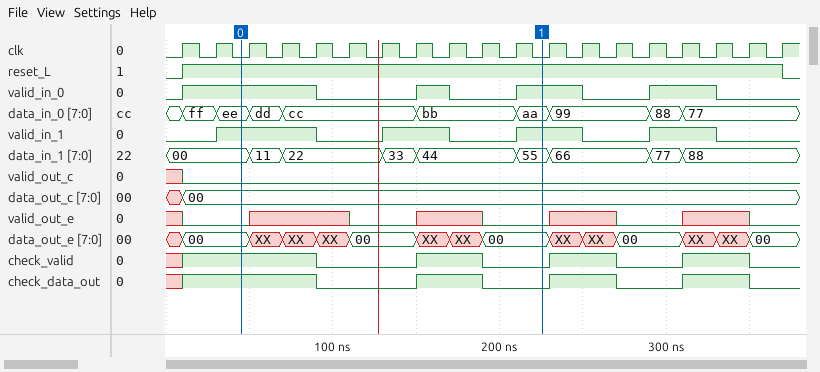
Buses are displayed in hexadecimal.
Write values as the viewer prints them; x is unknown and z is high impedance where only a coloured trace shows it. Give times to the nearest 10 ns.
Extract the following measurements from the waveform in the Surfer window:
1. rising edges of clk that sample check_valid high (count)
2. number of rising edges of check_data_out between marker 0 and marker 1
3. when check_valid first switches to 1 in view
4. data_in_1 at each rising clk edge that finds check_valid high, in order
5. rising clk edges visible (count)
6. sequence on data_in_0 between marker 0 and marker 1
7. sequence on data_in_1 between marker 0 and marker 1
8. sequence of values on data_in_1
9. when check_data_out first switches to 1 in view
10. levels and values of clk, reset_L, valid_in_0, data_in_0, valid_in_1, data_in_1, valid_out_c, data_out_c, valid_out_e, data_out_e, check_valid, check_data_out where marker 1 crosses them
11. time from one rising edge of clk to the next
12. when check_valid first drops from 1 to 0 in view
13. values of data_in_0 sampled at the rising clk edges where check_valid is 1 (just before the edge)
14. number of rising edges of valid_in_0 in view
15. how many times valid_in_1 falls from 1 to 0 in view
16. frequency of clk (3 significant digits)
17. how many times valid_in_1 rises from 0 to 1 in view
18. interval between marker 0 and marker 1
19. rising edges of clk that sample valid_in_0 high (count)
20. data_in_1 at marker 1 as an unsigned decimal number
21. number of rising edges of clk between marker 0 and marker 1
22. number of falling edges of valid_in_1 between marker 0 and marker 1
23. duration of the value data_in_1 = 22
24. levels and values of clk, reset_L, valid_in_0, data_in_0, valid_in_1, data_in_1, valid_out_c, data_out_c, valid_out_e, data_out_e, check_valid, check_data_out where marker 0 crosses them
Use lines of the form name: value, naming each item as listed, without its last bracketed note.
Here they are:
rising edges of clk that sample check_valid high: 10
number of rising edges of check_data_out between marker 0 and marker 1: 1
when check_valid first switches to 1 in view: 10 ns
data_in_1 at each rising clk edge that finds check_valid high, in order: 00, 00, 11, 22, 44, 44, 66, 66, 88, 88
rising clk edges visible: 19
sequence on data_in_0 between marker 0 and marker 1: ee, dd, cc, bb, aa
sequence on data_in_1 between marker 0 and marker 1: 00, 11, 22, 33, 44, 55
sequence of values on data_in_1: 00, 11, 22, 33, 44, 55, 66, 77, 88
when check_data_out first switches to 1 in view: 10 ns
levels and values of clk, reset_L, valid_in_0, data_in_0, valid_in_1, data_in_1, valid_out_c, data_out_c, valid_out_e, data_out_e, check_valid, check_data_out where marker 1 crosses them: clk=0, reset_L=1, valid_in_0=1, data_in_0=aa, valid_in_1=1, data_in_1=55, valid_out_c=0, data_out_c=00, valid_out_e=0, data_out_e=00, check_valid=0, check_data_out=0
time from one rising edge of clk to the next: 20 ns
when check_valid first drops from 1 to 0 in view: 90 ns
values of data_in_0 sampled at the rising clk edges where check_valid is 1: ff, ee, dd, cc, bb, bb, 99, 99, 77, 77
number of rising edges of valid_in_0 in view: 4
how many times valid_in_1 falls from 1 to 0 in view: 4
frequency of clk: 50.0 MHz
how many times valid_in_1 rises from 0 to 1 in view: 4
interval between marker 0 and marker 1: 180 ns
rising edges of clk that sample valid_in_0 high: 9
data_in_1 at marker 1 as an unsigned decimal number: 85
number of rising edges of clk between marker 0 and marker 1: 9
number of falling edges of valid_in_1 between marker 0 and marker 1: 2
duration of the value data_in_1 = 22: 60 ns
levels and values of clk, reset_L, valid_in_0, data_in_0, valid_in_1, data_in_1, valid_out_c, data_out_c, valid_out_e, data_out_e, check_valid, check_data_out where marker 0 crosses them: clk=0, reset_L=1, valid_in_0=1, data_in_0=ee, valid_in_1=1, data_in_1=00, valid_out_c=0, data_out_c=00, valid_out_e=0, data_out_e=00, check_valid=1, check_data_out=1
